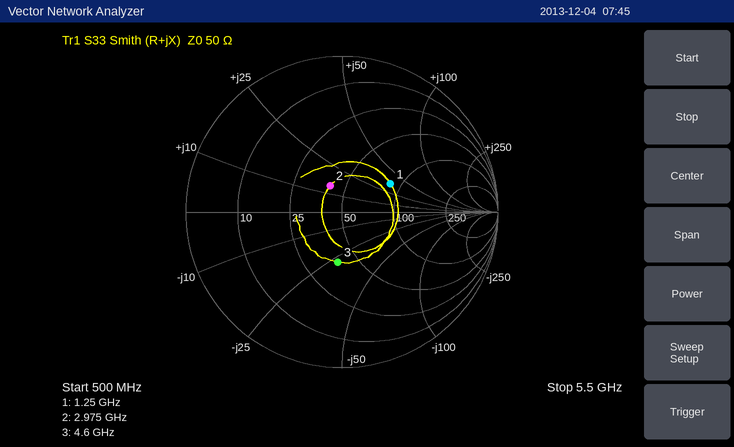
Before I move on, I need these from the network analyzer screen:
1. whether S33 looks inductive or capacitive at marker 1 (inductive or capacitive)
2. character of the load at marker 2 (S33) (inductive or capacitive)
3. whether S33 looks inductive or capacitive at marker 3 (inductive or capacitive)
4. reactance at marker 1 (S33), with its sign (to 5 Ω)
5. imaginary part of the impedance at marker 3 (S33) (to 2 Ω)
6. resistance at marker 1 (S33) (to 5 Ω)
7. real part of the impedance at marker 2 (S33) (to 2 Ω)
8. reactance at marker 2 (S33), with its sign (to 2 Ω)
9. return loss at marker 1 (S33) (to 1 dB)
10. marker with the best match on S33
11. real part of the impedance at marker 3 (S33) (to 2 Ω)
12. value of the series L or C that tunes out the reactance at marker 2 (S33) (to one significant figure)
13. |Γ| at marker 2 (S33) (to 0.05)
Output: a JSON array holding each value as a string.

["inductive", "inductive", "capacitive", "+35 Ω", "-28 Ω", "85 Ω", "40 Ω", "+14 Ω", "9 dB", "marker 2", "38 Ω", "4 pF", "0.20"]
